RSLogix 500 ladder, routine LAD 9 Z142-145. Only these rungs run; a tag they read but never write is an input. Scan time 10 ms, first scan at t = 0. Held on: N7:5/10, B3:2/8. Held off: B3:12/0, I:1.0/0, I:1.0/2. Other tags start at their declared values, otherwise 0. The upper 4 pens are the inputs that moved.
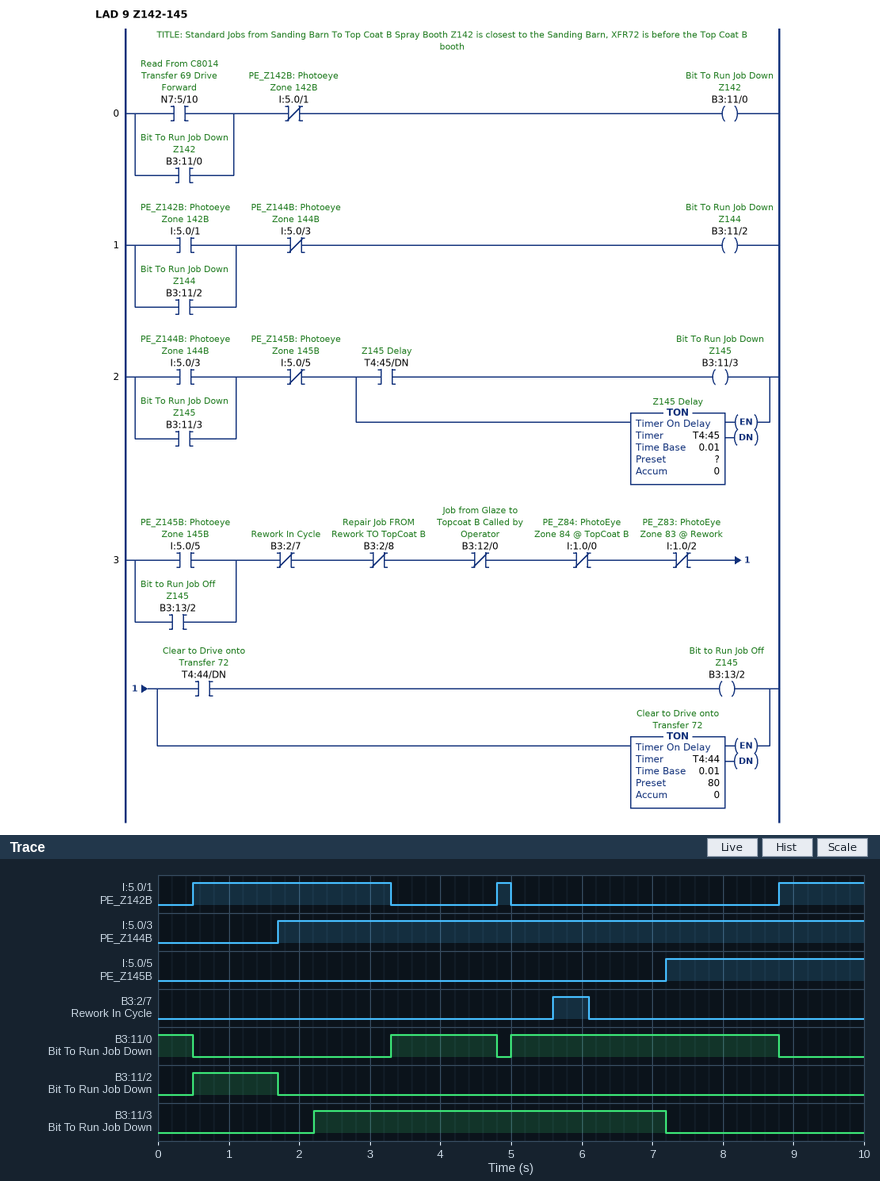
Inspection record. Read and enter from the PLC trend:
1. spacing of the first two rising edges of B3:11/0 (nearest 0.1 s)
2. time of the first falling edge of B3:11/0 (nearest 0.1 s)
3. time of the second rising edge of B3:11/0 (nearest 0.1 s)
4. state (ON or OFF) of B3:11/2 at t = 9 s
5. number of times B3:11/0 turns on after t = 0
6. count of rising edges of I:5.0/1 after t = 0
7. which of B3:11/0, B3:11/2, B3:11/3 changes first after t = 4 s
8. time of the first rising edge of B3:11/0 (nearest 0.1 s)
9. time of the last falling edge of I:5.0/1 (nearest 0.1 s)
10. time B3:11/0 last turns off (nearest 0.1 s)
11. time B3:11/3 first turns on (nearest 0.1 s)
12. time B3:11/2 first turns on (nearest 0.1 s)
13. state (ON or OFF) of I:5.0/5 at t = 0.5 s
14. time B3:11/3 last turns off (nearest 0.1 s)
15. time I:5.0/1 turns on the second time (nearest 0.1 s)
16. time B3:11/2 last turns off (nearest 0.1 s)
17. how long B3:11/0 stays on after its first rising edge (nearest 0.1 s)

1.7 s
0.5 s
5.0 s
OFF
2
3
B3:11/0
3.3 s
5.0 s
8.8 s
2.2 s
0.5 s
OFF
7.2 s
4.8 s
1.7 s
1.5 s
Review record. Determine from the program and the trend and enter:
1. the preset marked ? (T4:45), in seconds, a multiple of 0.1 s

0.5 s
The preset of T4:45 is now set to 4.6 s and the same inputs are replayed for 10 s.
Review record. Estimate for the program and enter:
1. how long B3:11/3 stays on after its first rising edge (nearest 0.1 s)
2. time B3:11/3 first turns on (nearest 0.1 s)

0.9 s
6.3 s
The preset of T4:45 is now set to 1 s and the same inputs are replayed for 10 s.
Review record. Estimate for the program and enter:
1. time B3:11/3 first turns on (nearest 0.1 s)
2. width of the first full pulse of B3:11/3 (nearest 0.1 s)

2.7 s
4.5 s
